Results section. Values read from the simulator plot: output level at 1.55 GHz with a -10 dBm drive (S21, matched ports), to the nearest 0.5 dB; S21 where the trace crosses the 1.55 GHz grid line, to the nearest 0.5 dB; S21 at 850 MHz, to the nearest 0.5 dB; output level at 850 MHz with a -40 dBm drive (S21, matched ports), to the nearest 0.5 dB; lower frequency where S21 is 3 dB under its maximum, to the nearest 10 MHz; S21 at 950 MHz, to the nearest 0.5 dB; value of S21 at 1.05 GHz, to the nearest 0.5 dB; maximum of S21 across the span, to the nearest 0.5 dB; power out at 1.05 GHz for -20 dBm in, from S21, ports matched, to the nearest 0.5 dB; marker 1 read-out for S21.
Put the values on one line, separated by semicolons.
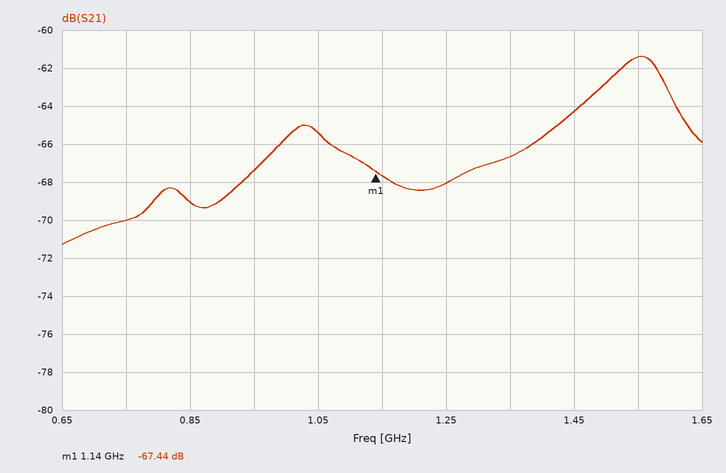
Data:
-71.5 dBm; -61.5 dB; -69.0 dB; -109.0 dBm; 1.45 GHz; -67.5 dB; -65.5 dB; -61.5 dB; -85.5 dBm; -67.44 dB
